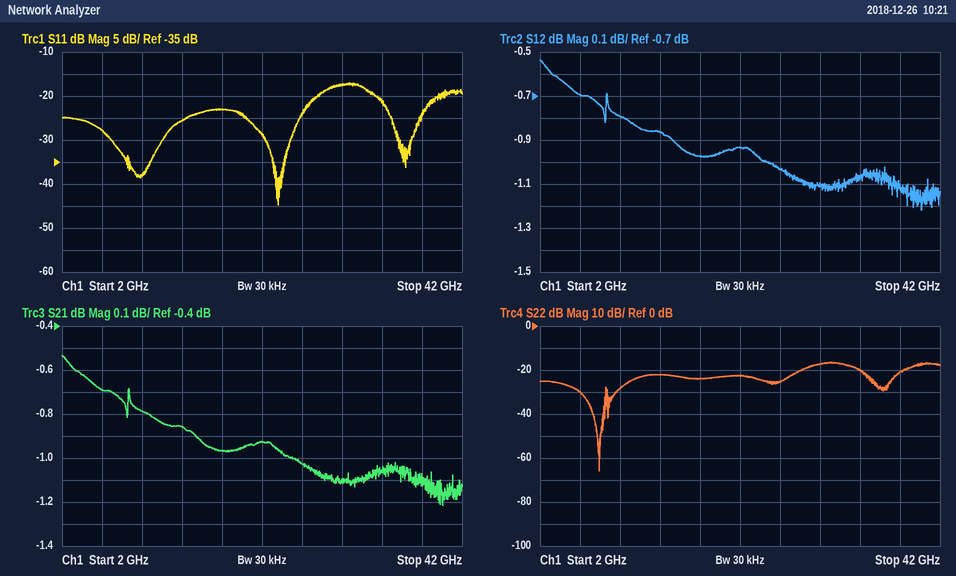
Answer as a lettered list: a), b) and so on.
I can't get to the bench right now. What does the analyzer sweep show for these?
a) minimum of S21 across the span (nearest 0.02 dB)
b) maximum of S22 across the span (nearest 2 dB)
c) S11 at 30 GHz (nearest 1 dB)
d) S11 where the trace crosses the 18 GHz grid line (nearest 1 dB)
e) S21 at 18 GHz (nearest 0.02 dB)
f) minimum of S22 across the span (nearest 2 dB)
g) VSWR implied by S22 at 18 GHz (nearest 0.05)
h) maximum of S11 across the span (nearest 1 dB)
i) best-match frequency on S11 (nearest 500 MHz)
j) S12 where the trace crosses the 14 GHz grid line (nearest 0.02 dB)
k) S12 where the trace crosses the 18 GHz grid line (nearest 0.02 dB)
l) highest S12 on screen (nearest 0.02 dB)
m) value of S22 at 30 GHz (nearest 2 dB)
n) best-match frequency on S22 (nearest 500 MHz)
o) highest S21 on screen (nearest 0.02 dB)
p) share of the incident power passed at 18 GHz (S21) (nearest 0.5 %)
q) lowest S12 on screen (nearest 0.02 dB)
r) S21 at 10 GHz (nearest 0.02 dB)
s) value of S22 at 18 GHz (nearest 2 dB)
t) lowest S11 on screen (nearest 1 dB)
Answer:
a) -1.22 dB
b) -16 dB
c) -17 dB
d) -23 dB
e) -0.96 dB
f) -66 dB
g) 1.15
h) -17 dB
i) 23.5 GHz
j) -0.86 dB
k) -0.98 dB
l) -0.54 dB
m) -18 dB
n) 8.0 GHz
o) -0.54 dB
p) 80.0 %
q) -1.22 dB
r) -0.78 dB
s) -24 dB
t) -45 dB
